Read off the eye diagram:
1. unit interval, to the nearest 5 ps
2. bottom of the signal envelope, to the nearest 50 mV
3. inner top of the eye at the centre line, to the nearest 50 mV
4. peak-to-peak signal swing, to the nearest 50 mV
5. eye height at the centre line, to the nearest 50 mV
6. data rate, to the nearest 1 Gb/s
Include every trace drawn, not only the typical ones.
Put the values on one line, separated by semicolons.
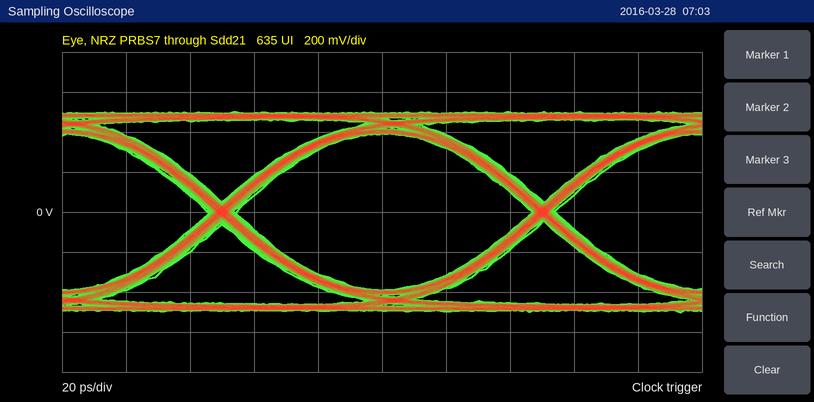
100 ps; -500 mV; 400 mV; 1.00 V; 800 mV; 10 Gb/s
